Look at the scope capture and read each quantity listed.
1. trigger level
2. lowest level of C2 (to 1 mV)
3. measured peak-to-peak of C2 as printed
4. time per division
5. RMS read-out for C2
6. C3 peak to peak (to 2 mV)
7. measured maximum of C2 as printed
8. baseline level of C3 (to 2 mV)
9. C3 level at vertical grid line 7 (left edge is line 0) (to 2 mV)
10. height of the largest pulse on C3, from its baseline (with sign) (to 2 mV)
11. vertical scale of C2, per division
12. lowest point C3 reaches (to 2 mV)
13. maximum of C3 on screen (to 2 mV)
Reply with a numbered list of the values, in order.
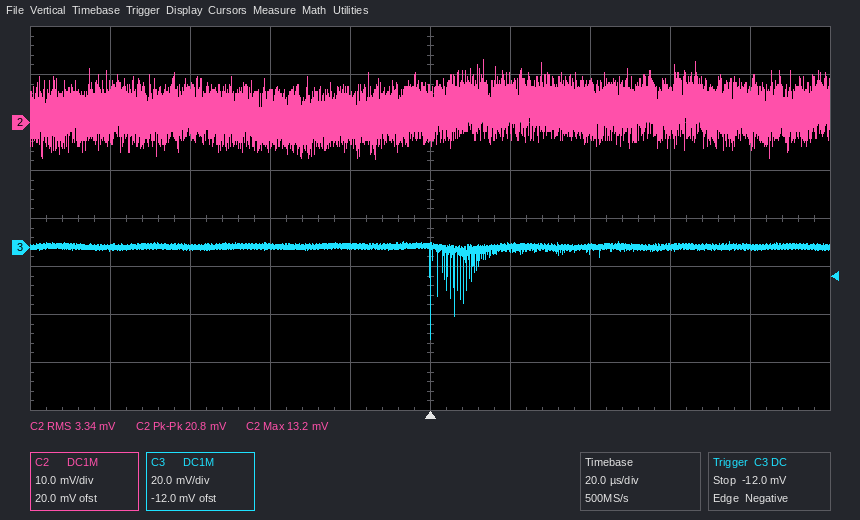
1. -12.0 mV
2. -8 mV
3. 20.8 mV
4. 20 µs
5. 3.34 mV
6. 40 mV
7. 13.2 mV
8. 0 mV
9. 0 mV
10. -38 mV
11. 10 mV
12. -38 mV
13. 2 mV
